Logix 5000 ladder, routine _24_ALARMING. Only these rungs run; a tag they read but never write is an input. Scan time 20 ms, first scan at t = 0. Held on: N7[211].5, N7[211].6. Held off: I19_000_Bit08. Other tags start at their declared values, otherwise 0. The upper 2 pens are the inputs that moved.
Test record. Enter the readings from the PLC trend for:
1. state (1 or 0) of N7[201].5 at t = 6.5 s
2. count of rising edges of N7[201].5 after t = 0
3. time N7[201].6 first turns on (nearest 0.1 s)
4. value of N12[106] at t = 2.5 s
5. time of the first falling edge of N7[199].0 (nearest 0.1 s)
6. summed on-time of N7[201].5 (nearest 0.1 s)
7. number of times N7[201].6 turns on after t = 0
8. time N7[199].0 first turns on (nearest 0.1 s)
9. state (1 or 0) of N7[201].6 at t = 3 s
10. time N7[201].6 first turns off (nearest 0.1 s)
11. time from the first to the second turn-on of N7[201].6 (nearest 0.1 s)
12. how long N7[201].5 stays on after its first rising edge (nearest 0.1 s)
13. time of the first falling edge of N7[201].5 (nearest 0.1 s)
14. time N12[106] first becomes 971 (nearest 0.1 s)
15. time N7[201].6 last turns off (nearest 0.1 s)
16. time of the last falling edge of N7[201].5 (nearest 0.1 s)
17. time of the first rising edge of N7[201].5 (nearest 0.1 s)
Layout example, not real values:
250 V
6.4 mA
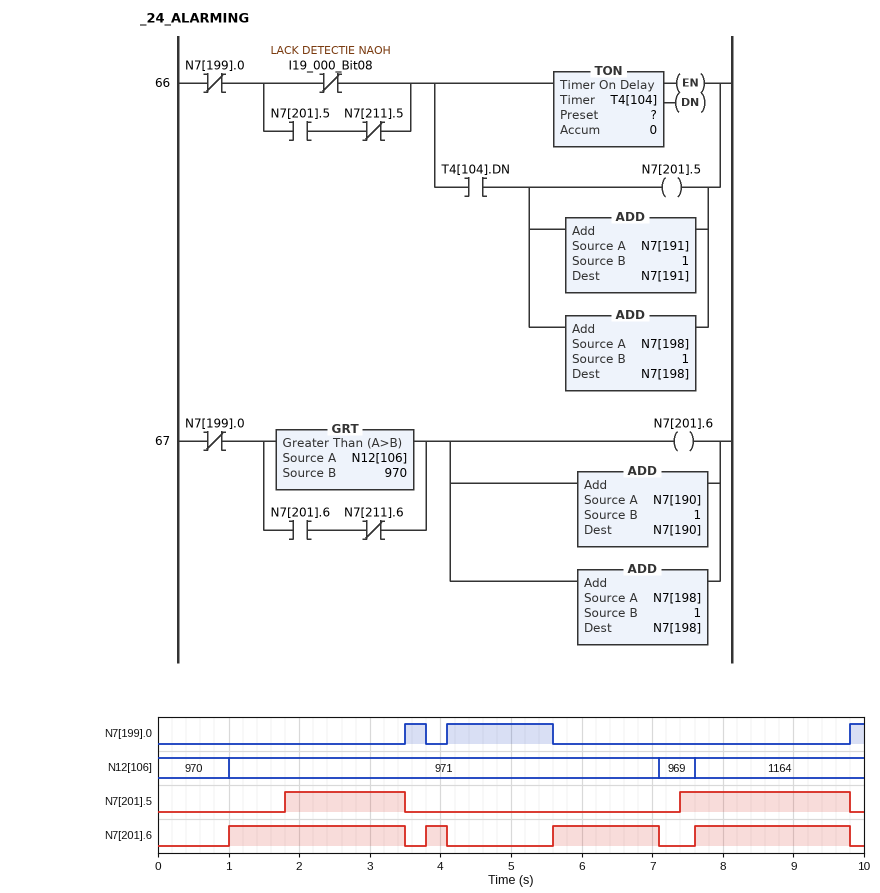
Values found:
0
2
1.0 s
971
3.8 s
4.1 s
4
3.5 s
1
3.5 s
2.8 s
1.7 s
3.5 s
1.0 s
9.8 s
9.8 s
1.8 s
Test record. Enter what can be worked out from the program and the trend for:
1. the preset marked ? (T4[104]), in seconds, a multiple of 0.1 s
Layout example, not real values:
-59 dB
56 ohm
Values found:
1.8 s
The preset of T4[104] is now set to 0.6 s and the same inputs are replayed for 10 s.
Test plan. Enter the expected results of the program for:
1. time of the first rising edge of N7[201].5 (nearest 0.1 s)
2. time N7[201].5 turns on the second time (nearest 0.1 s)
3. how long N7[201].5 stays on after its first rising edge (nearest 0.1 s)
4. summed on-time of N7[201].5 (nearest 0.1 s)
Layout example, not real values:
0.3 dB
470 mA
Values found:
0.6 s
6.2 s
2.9 s
6.5 s
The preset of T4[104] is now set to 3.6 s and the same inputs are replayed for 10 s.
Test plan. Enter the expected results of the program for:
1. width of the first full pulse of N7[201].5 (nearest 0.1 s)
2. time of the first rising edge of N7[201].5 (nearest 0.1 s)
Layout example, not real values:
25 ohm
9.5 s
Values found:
0.6 s
9.2 s
